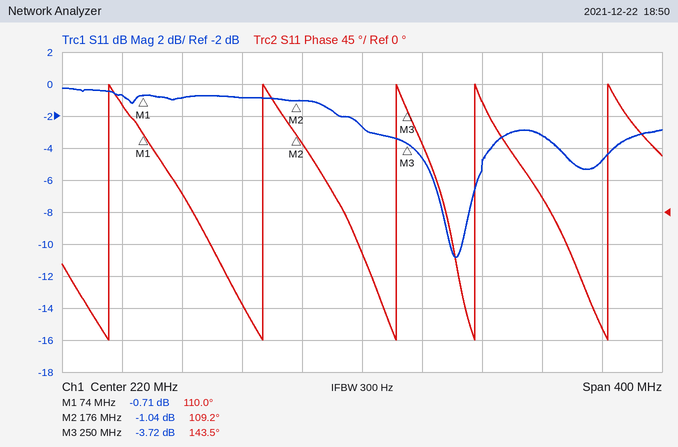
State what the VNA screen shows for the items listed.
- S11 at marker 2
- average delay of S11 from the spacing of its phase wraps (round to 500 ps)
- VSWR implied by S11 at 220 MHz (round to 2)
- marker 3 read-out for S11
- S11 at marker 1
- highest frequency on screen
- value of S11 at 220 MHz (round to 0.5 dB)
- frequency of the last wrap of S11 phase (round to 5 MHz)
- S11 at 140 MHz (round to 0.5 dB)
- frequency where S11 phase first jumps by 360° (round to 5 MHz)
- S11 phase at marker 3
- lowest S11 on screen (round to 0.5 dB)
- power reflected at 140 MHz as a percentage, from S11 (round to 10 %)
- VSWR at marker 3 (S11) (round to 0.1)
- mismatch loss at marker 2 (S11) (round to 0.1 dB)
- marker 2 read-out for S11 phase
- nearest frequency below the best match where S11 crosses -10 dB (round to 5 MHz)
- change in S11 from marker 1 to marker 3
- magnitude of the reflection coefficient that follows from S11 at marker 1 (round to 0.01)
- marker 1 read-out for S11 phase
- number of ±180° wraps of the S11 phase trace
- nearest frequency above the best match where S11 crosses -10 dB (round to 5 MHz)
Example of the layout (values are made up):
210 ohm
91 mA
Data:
-1.04 dB
12.0 ns
6
-3.72 dB
-0.71 dB
420 MHz
-2.5 dB
385 MHz
-1.0 dB
50 MHz
143.5°
-11.0 dB
80 %
4.7
6.7 dB
109.2°
280 MHz
-3.01 dB
0.92
110.0°
5
285 MHz
